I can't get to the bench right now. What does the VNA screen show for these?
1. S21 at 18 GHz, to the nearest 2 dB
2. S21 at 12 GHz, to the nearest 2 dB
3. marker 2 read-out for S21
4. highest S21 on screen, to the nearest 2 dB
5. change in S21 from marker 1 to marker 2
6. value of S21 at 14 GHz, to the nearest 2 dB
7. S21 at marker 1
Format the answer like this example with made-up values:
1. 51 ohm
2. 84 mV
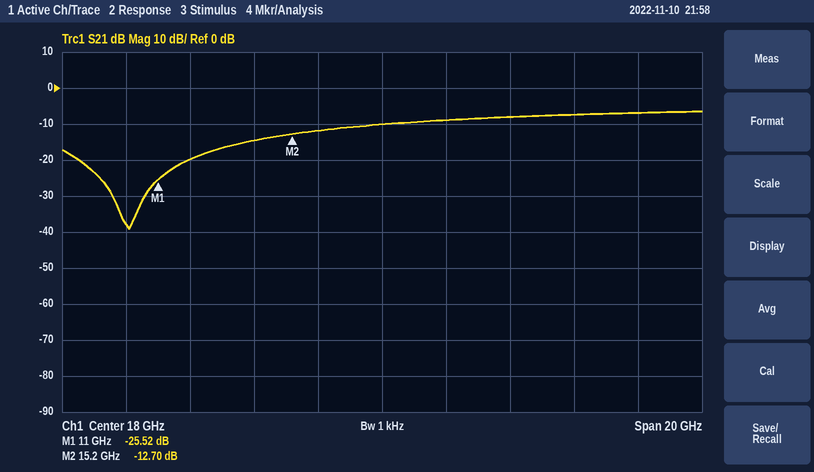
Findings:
1. -10 dB
2. -20 dB
3. -12.70 dB
4. -6 dB
5. 12.82 dB
6. -14 dB
7. -25.52 dB
